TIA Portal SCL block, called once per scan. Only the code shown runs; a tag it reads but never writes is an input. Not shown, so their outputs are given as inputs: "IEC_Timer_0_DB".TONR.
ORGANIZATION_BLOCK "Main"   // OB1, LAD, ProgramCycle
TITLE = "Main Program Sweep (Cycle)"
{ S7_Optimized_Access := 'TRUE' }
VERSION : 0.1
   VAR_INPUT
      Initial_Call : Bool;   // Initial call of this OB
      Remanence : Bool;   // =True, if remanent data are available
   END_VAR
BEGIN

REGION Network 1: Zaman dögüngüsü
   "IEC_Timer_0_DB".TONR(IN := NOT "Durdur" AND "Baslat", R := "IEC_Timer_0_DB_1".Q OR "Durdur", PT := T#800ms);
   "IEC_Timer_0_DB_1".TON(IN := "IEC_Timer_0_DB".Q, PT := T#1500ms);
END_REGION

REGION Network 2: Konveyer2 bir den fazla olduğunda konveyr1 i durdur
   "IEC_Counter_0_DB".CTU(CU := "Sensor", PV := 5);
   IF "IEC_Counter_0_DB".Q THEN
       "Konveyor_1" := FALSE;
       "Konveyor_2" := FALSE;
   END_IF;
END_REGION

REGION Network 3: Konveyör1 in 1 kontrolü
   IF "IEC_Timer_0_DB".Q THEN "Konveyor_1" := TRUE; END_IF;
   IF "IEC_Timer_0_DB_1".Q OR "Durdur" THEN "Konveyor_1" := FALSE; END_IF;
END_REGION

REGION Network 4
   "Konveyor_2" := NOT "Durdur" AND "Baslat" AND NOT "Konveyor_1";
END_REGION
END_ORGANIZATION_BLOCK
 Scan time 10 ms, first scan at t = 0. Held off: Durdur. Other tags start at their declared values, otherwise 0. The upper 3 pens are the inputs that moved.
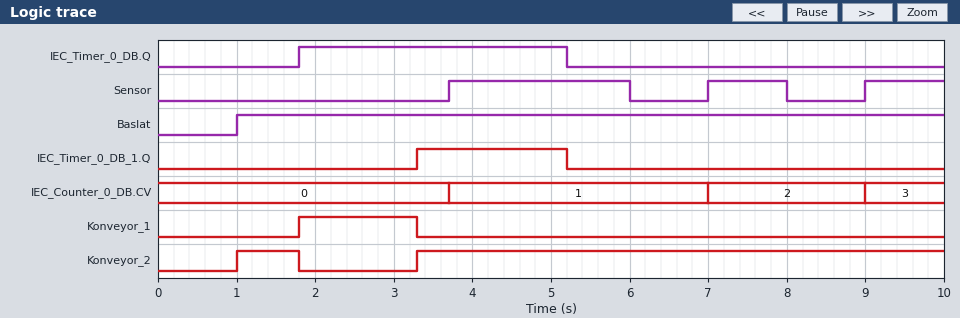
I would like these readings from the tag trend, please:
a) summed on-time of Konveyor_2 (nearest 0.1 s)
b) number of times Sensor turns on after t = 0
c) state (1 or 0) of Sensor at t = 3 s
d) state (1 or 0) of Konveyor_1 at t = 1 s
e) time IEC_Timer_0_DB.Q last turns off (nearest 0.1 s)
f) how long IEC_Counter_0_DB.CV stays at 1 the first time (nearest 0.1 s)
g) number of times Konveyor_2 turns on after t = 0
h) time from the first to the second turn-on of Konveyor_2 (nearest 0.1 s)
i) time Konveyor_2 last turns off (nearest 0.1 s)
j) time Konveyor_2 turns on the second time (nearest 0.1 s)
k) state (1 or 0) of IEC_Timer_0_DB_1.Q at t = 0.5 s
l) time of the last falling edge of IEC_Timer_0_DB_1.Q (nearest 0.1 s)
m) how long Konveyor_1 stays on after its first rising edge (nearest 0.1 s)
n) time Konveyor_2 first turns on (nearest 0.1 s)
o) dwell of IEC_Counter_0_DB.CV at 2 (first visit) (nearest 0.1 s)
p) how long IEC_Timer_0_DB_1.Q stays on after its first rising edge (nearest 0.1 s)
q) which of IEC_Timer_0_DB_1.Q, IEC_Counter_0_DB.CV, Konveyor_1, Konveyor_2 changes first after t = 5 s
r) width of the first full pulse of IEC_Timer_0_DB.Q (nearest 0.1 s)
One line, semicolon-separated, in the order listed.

7.5 s; 3; 0; 0; 5.2 s; 3.3 s; 2; 2.3 s; 1.8 s; 3.3 s; 0; 5.2 s; 1.5 s; 1.0 s; 2.0 s; 1.9 s; IEC_Timer_0_DB_1.Q; 3.4 s
